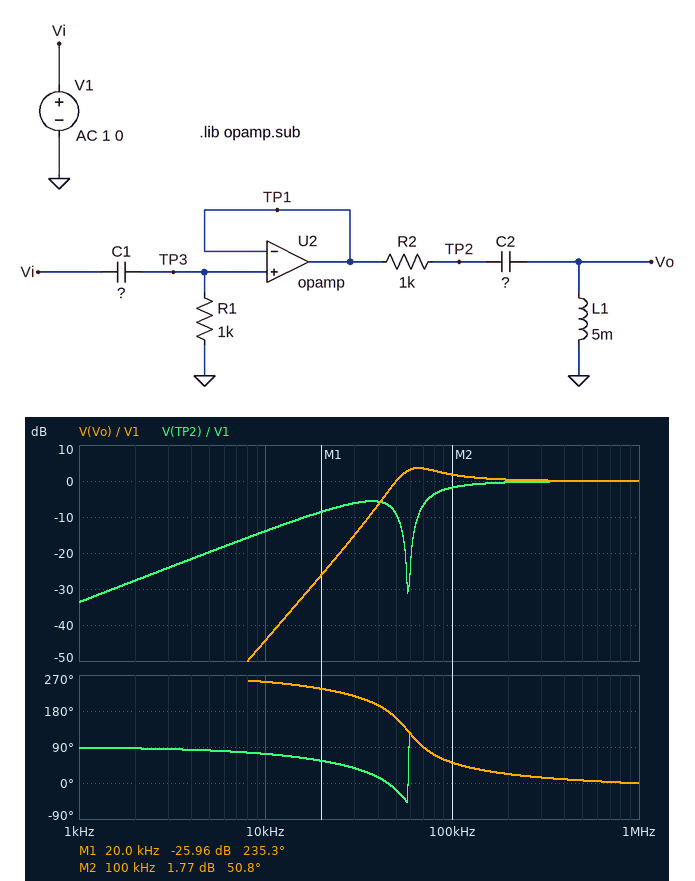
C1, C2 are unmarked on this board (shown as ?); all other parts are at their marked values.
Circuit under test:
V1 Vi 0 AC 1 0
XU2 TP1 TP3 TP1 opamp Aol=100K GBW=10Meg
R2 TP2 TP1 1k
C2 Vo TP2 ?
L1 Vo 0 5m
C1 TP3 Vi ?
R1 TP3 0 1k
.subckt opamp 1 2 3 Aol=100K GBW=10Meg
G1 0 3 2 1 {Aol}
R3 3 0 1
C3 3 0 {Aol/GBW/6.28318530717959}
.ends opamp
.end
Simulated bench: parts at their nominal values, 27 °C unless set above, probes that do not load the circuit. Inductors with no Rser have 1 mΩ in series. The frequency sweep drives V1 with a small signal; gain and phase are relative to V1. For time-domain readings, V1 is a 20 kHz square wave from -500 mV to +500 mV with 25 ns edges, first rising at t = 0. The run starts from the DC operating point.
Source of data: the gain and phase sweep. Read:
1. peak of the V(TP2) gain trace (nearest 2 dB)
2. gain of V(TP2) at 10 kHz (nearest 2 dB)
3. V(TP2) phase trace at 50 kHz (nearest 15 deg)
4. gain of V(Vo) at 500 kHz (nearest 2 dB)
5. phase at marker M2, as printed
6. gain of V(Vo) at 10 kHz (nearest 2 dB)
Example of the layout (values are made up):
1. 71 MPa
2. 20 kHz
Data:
1. 0 dB
2. -14 dB
3. -15 deg
4. 0 dB
5. 50.8 deg
6. -44 dB
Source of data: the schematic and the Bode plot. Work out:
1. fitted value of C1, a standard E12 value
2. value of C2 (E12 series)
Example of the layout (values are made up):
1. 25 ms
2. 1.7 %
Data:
1. 3.3 nF
2. 1.5 nF
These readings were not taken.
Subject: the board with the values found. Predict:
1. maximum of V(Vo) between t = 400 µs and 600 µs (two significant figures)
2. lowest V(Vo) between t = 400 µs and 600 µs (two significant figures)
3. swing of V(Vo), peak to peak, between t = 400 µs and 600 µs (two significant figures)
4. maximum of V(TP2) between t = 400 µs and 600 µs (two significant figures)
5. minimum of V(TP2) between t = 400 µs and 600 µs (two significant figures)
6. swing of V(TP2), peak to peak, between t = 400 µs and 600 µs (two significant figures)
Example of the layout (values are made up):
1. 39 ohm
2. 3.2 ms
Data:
1. 1.0 V
2. -1.0 V
3. 2.1 V
4. 960 mV
5. -960 mV
6. 1.9 V
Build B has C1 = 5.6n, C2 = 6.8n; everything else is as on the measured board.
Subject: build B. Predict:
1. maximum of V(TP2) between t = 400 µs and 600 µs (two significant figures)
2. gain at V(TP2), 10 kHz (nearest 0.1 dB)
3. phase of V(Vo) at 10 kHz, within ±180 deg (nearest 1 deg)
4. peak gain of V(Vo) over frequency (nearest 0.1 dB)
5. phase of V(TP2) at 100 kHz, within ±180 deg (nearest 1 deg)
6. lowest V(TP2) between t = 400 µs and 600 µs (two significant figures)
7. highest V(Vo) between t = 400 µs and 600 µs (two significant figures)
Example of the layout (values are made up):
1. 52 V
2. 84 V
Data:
1. 810 mV
2. -10.5 dB
3. -136 deg
4. 0 dB
5. 34 deg
6. -810 mV
7. 900 mV
